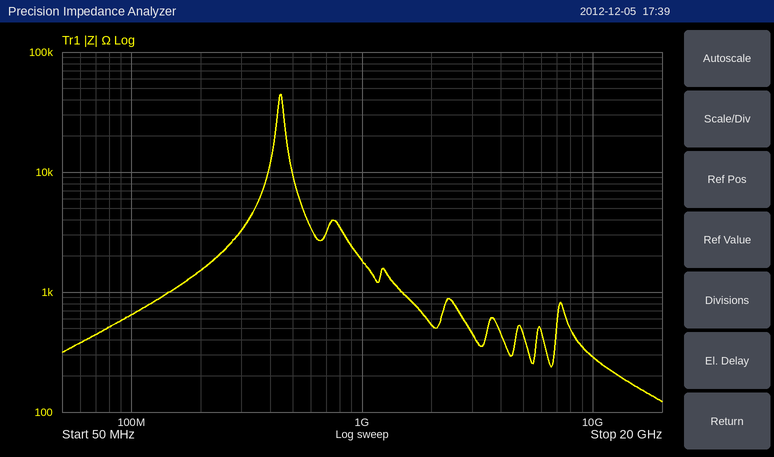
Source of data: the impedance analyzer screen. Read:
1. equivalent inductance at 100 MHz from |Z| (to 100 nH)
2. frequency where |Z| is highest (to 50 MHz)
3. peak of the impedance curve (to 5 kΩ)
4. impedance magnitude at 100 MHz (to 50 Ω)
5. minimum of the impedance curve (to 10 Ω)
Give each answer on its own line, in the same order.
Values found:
1.0 µH
450 MHz
45 kΩ
650 Ω
120 Ω
